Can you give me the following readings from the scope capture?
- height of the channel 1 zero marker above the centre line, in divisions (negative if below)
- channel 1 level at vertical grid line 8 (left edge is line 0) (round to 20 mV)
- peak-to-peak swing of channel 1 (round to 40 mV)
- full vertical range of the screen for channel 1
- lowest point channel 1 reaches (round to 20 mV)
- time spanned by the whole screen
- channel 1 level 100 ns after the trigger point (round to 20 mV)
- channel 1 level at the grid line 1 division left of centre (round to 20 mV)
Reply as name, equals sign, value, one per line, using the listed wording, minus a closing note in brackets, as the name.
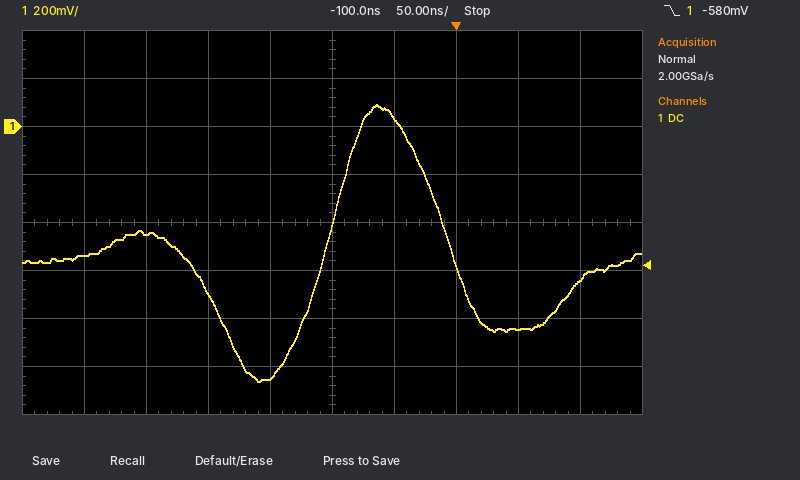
height of the channel 1 zero marker above the centre line, in divisions = +2.0 div
channel 1 level at vertical grid line 8 (left edge is line 0) = -840 mV
peak-to-peak swing of channel 1 = 1.16 V
full vertical range of the screen for channel 1 = 1.6 V
lowest point channel 1 reaches = -1.06 V
time spanned by the whole screen = 500 ns
channel 1 level 100 ns after the trigger point = -640 mV
channel 1 level at the grid line 1 division left of centre = -1.04 V
